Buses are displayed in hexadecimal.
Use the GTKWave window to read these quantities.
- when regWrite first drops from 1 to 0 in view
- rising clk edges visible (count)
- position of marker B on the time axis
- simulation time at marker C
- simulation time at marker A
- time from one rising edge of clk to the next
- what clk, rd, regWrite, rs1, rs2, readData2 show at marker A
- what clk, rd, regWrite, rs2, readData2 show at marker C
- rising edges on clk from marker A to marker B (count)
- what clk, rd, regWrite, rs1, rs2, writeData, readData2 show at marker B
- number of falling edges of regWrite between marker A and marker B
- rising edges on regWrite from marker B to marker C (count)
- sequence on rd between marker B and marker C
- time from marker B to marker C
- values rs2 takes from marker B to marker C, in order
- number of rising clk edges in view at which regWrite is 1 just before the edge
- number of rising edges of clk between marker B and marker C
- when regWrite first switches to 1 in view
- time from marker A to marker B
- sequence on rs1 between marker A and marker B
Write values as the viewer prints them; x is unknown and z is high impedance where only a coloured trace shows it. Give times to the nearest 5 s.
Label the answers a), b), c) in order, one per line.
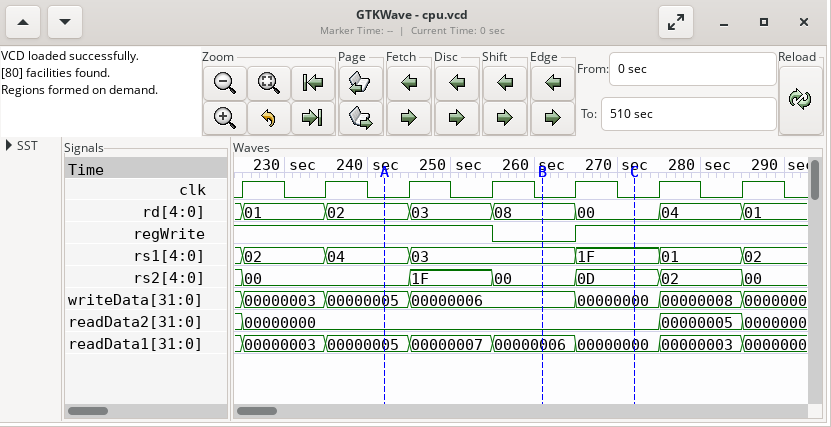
a) 255 s
b) 7
c) 260 s
d) 270 s
e) 240 s
f) 10 s
g) clk=0, rd=02, regWrite=1, rs1=04, rs2=00, readData2=00000000
h) clk=0, rd=00, regWrite=1, rs2=0D, readData2=00000000
i) 2
j) clk=0, rd=08, regWrite=0, rs1=03, rs2=00, writeData=00000006, readData2=00000000
k) 1
l) 1
m) 08, 00
n) 10 s
o) 00, 0D
p) 6
q) 1
r) 265 s
s) 20 s
t) 04, 03
